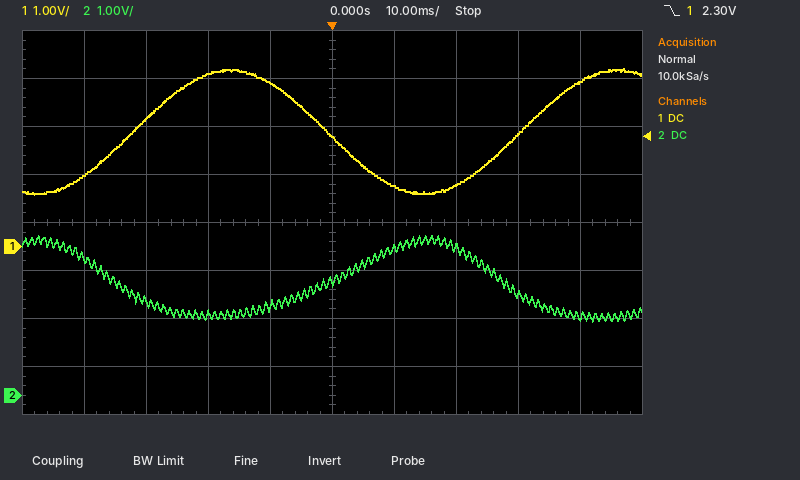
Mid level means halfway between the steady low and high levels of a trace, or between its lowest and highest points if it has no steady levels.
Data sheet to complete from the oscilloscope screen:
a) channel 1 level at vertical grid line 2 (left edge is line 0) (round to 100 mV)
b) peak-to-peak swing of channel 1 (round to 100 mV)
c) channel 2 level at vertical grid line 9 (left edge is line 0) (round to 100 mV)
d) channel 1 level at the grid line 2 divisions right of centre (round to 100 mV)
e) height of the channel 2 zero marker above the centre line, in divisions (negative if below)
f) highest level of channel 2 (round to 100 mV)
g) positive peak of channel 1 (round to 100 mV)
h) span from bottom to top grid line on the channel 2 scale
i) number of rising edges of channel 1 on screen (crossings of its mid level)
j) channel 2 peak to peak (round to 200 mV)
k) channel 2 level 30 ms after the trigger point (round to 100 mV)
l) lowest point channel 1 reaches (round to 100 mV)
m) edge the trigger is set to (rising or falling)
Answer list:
2.7 V
2.6 V
1.7 V
1.3 V
-3.6 div
3.3 V
3.7 V
8 V
2
1.8 V
2.1 V
1.1 V
falling
